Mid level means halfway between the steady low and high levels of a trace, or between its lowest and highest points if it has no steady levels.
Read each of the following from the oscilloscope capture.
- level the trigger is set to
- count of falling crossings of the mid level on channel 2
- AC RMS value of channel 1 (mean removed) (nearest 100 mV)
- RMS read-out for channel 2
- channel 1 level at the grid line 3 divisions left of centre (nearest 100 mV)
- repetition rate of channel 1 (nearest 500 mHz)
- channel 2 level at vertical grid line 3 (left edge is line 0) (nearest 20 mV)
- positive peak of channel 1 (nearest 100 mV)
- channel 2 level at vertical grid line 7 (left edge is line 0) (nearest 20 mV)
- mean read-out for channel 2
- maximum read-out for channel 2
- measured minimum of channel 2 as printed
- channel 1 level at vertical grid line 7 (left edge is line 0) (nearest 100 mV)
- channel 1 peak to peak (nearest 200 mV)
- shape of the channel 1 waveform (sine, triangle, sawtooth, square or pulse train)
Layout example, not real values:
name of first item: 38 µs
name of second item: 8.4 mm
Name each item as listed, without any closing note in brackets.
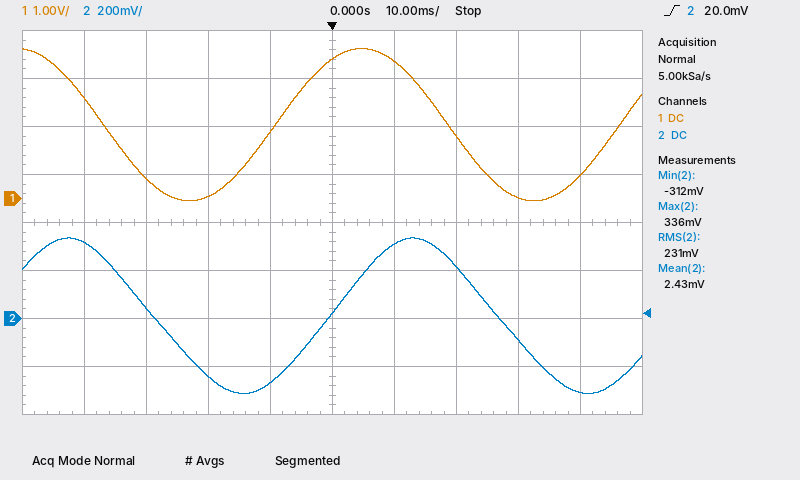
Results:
level the trigger is set to: 20.0 mV
count of falling crossings of the mid level on channel 2: 2
AC RMS value of channel 1 (mean removed): 1.1 V
RMS read-out for channel 2: 231 mV
channel 1 level at the grid line 3 divisions left of centre: 400 mV
repetition rate of channel 1: 18.0 Hz
channel 2 level at vertical grid line 3 (left edge is line 0): -240 mV
positive peak of channel 1: 3.1 V
channel 2 level at vertical grid line 7 (left edge is line 0): 220 mV
mean read-out for channel 2: 2.43 mV
maximum read-out for channel 2: 336 mV
measured minimum of channel 2 as printed: -312 mV
channel 1 level at vertical grid line 7 (left edge is line 0): 1.3 V
channel 1 peak to peak: 3.2 V
shape of the channel 1 waveform: sine
